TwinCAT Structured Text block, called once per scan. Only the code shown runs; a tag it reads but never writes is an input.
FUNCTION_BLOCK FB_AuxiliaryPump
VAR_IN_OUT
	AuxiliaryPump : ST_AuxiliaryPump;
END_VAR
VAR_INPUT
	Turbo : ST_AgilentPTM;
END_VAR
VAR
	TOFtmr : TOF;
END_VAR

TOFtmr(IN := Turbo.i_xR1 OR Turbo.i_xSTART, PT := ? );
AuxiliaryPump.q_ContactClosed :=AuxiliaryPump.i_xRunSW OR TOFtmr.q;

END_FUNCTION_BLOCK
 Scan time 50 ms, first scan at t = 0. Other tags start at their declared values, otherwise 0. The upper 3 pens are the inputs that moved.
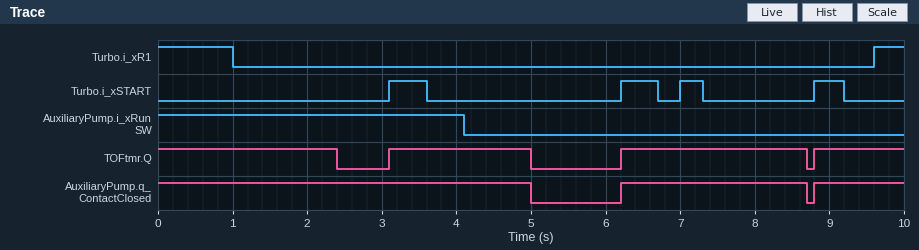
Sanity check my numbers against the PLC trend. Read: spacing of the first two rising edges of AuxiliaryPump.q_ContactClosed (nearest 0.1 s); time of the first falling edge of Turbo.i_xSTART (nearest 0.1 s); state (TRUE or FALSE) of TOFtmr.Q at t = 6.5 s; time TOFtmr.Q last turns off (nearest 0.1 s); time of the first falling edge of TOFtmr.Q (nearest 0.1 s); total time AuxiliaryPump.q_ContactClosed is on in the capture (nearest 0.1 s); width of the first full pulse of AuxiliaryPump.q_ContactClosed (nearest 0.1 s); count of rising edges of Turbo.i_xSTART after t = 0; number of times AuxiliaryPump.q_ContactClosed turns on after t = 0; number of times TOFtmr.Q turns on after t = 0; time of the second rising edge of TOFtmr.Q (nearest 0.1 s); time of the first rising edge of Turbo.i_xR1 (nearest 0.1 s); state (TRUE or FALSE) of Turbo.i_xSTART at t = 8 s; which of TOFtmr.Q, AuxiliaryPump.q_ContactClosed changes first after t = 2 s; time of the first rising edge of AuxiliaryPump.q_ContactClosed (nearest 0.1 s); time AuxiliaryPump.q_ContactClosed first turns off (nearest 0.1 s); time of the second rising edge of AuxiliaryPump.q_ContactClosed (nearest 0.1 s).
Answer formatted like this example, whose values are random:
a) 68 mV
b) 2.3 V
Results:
a) 2.6 s
b) 3.6 s
c) TRUE
d) 8.7 s
e) 2.4 s
f) 8.7 s
g) 2.5 s
h) 4
i) 2
j) 3
k) 6.2 s
l) 9.6 s
m) FALSE
n) TOFtmr.Q
o) 6.2 s
p) 5.0 s
q) 8.8 s
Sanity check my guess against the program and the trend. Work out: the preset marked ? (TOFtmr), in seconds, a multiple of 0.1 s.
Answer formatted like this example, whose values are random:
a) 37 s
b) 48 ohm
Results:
a) 1.4 s
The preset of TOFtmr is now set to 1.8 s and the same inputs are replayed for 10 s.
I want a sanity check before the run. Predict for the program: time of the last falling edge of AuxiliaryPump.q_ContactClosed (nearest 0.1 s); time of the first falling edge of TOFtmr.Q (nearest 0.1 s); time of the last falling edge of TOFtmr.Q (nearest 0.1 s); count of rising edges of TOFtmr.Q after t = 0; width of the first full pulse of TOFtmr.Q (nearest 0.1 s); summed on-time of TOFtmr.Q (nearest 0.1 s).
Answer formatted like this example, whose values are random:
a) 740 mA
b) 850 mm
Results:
a) 5.4 s
b) 2.8 s
c) 5.4 s
d) 2
e) 2.3 s
f) 8.9 s
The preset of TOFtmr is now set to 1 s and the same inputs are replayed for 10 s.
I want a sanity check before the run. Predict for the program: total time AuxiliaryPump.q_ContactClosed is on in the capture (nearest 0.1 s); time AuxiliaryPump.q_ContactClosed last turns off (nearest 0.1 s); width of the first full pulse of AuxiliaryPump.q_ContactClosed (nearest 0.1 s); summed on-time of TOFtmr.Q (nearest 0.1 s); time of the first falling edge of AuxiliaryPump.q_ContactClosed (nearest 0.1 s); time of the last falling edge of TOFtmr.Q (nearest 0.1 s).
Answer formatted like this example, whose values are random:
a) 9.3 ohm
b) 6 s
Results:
a) 7.9 s
b) 8.3 s
c) 2.1 s
d) 6.8 s
e) 4.6 s
f) 8.3 s
